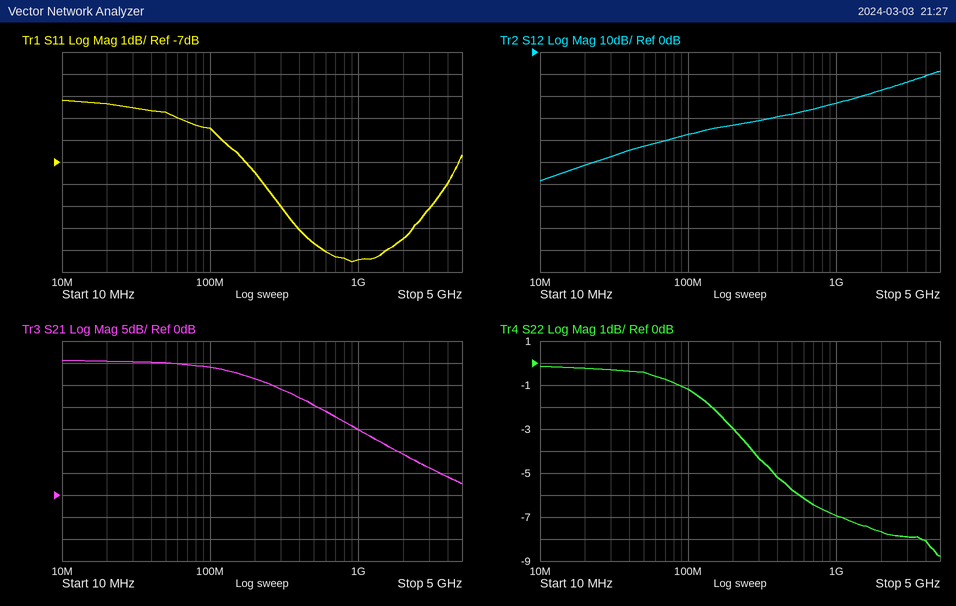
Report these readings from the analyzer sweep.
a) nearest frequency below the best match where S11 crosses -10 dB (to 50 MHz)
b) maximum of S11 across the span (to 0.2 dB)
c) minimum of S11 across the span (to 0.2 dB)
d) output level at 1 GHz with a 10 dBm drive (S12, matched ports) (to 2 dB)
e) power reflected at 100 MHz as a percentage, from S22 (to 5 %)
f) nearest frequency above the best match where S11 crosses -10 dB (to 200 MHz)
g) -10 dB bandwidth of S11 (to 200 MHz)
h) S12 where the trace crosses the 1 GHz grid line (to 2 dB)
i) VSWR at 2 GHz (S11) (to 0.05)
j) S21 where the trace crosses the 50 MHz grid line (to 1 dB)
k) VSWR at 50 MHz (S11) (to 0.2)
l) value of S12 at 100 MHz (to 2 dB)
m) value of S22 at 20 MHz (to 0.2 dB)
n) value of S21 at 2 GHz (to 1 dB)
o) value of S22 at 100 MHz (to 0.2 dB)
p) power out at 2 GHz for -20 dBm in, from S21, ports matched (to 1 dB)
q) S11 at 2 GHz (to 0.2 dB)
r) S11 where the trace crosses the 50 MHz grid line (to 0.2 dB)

400 MHz
-4.2 dB
-11.6 dB
-14 dBm
75 %
2.4 GHz
2.0 GHz
-24 dB
1.85
30 dB
3.8
-38 dB
-0.2 dB
9 dB
-1.2 dB
-11 dBm
-10.4 dB
-4.8 dB
